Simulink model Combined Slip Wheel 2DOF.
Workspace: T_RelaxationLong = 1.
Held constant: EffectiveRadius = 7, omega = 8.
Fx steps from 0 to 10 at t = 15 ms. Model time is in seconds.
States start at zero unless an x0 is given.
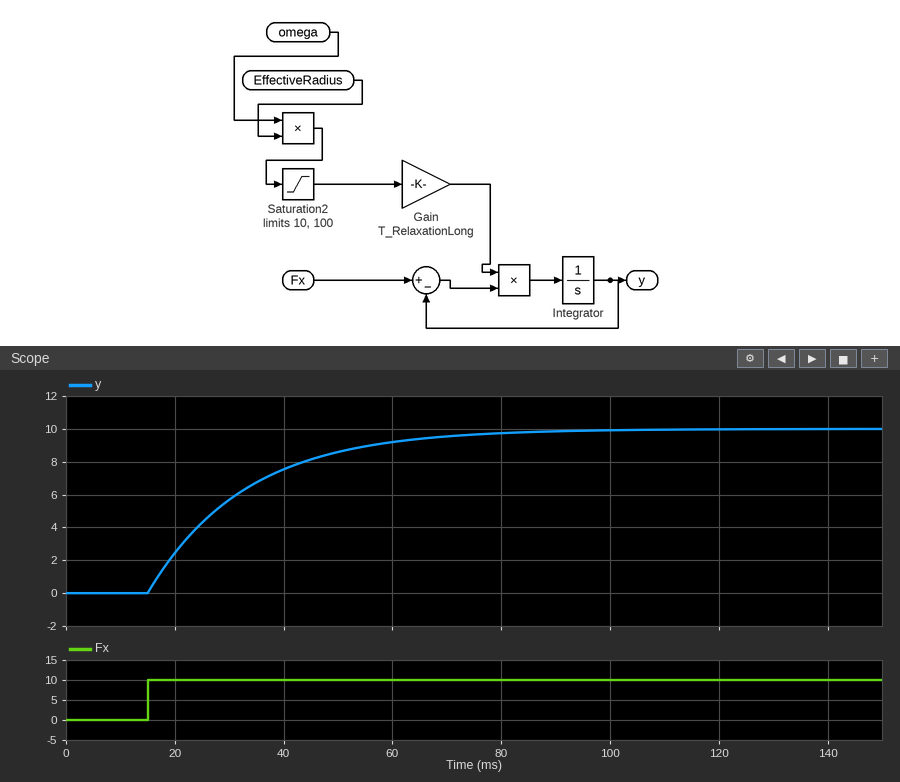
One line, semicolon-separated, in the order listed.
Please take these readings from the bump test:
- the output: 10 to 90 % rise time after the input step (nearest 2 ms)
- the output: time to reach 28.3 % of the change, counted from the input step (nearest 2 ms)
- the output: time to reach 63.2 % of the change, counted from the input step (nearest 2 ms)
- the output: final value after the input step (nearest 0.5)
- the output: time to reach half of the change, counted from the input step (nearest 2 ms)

40 ms; 6 ms; 18 ms; 10.0; 12 ms
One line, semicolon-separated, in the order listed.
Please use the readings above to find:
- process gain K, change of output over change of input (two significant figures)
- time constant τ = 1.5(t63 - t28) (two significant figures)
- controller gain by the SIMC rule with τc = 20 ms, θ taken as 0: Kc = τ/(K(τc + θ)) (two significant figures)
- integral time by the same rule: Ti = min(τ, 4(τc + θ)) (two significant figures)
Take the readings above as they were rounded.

1.0; 18 ms; 0.90; 18 ms
